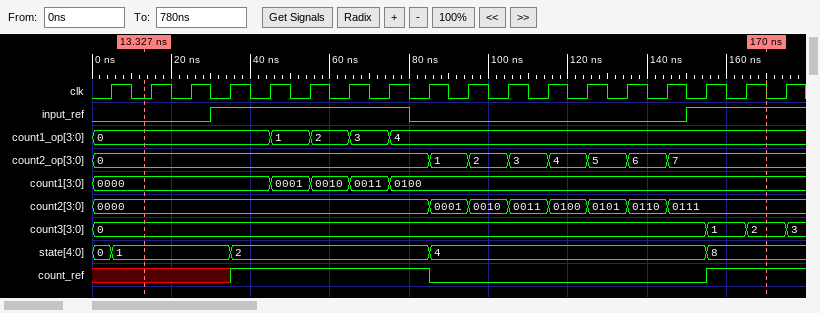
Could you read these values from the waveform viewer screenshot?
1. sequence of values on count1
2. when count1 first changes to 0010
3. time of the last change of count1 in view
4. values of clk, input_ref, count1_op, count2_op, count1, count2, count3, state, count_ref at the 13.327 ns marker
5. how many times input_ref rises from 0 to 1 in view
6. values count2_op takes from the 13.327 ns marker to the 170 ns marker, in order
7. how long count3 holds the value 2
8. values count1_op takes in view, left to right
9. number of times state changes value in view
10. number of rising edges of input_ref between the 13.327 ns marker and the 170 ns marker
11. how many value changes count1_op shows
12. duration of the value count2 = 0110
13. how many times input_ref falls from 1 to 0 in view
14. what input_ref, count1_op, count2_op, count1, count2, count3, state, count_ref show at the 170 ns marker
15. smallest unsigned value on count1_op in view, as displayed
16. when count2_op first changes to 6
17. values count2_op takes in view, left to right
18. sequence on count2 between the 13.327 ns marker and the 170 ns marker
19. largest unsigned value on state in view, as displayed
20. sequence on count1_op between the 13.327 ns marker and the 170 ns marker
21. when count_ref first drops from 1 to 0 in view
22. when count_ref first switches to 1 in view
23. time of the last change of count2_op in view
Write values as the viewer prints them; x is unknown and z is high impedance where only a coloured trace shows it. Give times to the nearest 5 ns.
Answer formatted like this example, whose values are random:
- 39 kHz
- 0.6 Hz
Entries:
- 0000, 0001, 0010, 0011, 0100
- 55 ns
- 75 ns
- clk=0, input_ref=0, count1_op=0, count2_op=0, count1=0000, count2=0000, count3=0, state=1, count_ref=x
- 2
- 0, 1, 2, 3, 4, 5, 6, 7
- 10 ns
- 0, 1, 2, 3, 4
- 4
- 2
- 4
- 10 ns
- 1
- input_ref=1, count1_op=4, count2_op=7, count1=0100, count2=0111, count3=2, state=8, count_ref=1
- 0
- 135 ns
- 0, 1, 2, 3, 4, 5, 6, 7
- 0000, 0001, 0010, 0011, 0100, 0101, 0110, 0111
- 8
- 0, 1, 2, 3, 4
- 85 ns
- 35 ns
- 145 ns
